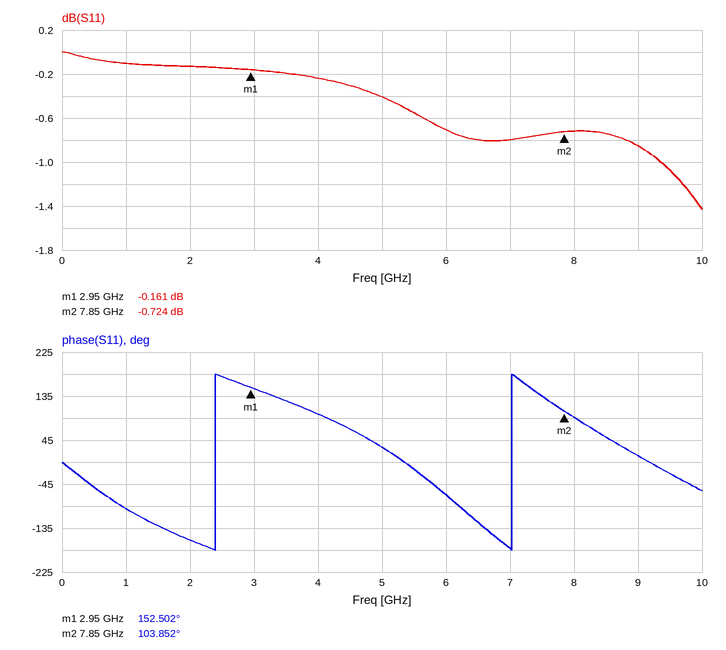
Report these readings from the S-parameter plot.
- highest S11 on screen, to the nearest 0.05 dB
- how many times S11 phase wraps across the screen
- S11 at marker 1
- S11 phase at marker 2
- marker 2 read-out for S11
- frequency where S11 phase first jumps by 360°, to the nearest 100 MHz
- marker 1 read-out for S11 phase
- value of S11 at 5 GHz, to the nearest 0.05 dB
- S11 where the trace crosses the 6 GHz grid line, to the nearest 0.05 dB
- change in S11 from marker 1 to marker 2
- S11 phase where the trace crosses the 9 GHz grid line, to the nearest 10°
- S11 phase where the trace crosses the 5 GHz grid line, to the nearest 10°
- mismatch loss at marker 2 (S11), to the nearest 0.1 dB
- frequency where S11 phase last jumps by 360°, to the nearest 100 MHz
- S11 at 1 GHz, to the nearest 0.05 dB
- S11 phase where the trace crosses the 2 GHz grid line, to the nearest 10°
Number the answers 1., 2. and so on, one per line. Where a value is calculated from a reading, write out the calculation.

1. 0.00 dB
2. 2
3. -0.161 dB
4. 103.852°
5. -0.724 dB
6. 2.4 GHz
7. 152.502°
8. -0.40 dB
9. -0.70 dB
10. -0.724 − (-0.161) = -0.563 dB
11. 10°
12. 30°
13. −10 log10(1 − 10^(-0.724/10)) ≈ 8.1 dB
14. 7.0 GHz
15. -0.10 dB
16. -160°
